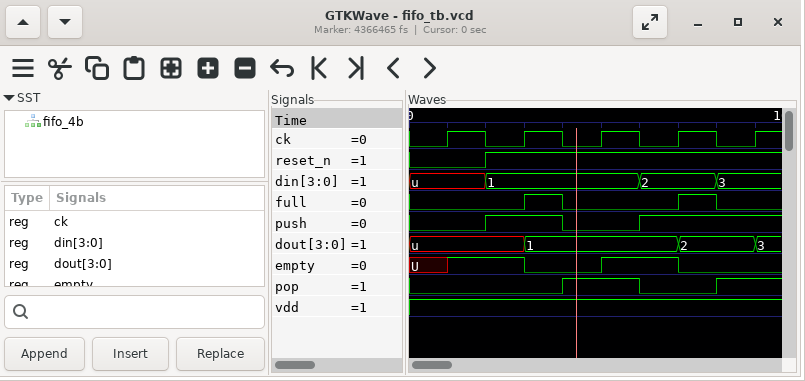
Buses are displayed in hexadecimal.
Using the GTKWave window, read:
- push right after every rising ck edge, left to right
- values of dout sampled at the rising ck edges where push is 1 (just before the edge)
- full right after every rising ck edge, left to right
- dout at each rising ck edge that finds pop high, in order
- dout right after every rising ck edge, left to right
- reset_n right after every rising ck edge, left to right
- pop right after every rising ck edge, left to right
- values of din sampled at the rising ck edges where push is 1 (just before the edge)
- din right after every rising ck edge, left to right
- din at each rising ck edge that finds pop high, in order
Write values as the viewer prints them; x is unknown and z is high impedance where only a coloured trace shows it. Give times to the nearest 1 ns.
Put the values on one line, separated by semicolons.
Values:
0 1 0 1 1; u, 1, 2; 0 1 0 1 0; 1, 2; u, 1, 1, 2, 3; 0 1 1 1 1; 0 0 1 0 1; 1, 2, 3; u, 1, 1, 2, 3; 1, 3
